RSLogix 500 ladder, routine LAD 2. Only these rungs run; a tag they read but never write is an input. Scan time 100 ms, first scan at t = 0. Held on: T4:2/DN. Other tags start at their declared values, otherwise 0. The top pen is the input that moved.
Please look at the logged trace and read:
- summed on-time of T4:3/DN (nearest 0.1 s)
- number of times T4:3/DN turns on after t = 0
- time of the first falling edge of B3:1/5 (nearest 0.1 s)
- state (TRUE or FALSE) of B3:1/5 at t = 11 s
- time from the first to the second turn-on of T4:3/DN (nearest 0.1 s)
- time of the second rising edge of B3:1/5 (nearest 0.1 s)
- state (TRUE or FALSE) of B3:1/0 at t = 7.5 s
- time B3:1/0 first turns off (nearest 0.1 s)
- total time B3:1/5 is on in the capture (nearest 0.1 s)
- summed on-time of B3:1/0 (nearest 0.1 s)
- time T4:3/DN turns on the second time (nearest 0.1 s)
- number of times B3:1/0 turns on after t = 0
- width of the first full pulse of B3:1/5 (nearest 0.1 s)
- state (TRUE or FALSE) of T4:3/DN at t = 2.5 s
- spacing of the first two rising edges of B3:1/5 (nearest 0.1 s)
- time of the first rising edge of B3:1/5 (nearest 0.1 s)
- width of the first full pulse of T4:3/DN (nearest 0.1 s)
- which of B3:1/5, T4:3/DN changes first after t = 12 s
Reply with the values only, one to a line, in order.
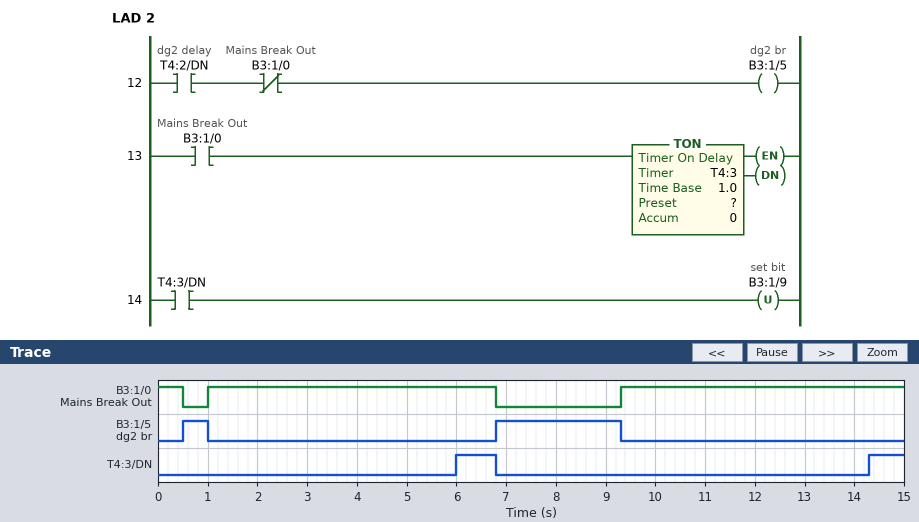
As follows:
1.5 s
2
1.0 s
FALSE
8.3 s
6.8 s
FALSE
0.5 s
3.0 s
12.0 s
14.3 s
2
0.5 s
FALSE
6.3 s
0.5 s
0.8 s
T4:3/DN
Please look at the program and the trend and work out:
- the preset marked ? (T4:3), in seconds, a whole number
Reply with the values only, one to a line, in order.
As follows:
5 s
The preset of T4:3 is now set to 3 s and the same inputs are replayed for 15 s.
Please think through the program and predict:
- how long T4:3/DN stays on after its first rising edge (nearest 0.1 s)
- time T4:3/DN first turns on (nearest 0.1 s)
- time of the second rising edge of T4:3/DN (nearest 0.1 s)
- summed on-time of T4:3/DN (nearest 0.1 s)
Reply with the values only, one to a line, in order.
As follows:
2.8 s
4.0 s
12.3 s
5.5 s
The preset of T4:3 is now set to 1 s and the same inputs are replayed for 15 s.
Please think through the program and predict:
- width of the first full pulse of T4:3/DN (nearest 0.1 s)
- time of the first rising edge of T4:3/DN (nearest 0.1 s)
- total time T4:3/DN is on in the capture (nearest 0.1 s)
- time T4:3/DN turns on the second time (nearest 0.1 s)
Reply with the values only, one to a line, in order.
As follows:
4.8 s
2.0 s
9.5 s
10.3 s
